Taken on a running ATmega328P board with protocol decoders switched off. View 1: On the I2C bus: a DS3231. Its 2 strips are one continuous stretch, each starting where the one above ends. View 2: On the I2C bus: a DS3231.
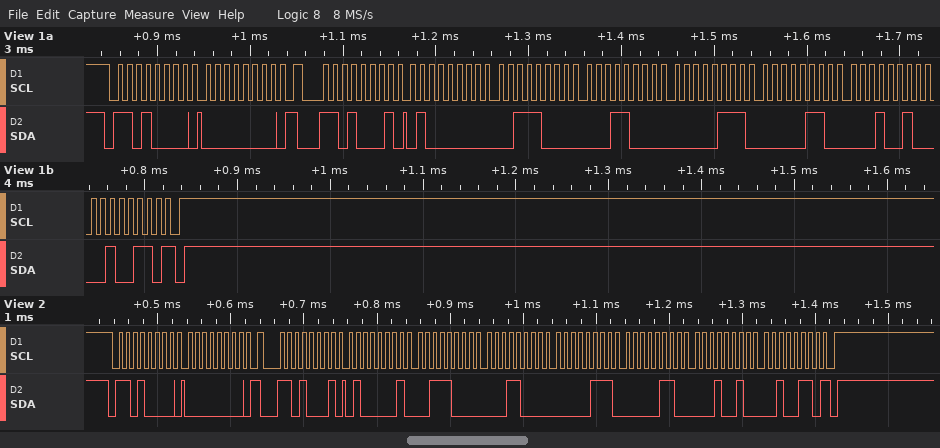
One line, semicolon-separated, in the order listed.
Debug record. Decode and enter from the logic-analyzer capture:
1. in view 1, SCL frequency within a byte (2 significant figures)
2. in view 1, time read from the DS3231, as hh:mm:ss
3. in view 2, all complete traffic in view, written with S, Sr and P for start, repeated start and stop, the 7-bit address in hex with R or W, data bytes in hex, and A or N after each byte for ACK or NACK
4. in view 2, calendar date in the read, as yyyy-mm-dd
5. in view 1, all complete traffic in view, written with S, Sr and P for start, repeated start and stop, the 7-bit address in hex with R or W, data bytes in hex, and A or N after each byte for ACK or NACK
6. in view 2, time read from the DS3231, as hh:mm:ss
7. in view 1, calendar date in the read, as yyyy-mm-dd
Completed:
100 kHz; 18:38:40; S 68W A 00 A Sr 68R A 41 A 38 A 18 A 07 A 06 A 12 A 26 N P; 2026-12-06; S 68W A 00 A Sr 68R A 40 A 38 A 18 A 07 A 06 A 12 A 26 N P; 18:38:41; 2026-12-06
